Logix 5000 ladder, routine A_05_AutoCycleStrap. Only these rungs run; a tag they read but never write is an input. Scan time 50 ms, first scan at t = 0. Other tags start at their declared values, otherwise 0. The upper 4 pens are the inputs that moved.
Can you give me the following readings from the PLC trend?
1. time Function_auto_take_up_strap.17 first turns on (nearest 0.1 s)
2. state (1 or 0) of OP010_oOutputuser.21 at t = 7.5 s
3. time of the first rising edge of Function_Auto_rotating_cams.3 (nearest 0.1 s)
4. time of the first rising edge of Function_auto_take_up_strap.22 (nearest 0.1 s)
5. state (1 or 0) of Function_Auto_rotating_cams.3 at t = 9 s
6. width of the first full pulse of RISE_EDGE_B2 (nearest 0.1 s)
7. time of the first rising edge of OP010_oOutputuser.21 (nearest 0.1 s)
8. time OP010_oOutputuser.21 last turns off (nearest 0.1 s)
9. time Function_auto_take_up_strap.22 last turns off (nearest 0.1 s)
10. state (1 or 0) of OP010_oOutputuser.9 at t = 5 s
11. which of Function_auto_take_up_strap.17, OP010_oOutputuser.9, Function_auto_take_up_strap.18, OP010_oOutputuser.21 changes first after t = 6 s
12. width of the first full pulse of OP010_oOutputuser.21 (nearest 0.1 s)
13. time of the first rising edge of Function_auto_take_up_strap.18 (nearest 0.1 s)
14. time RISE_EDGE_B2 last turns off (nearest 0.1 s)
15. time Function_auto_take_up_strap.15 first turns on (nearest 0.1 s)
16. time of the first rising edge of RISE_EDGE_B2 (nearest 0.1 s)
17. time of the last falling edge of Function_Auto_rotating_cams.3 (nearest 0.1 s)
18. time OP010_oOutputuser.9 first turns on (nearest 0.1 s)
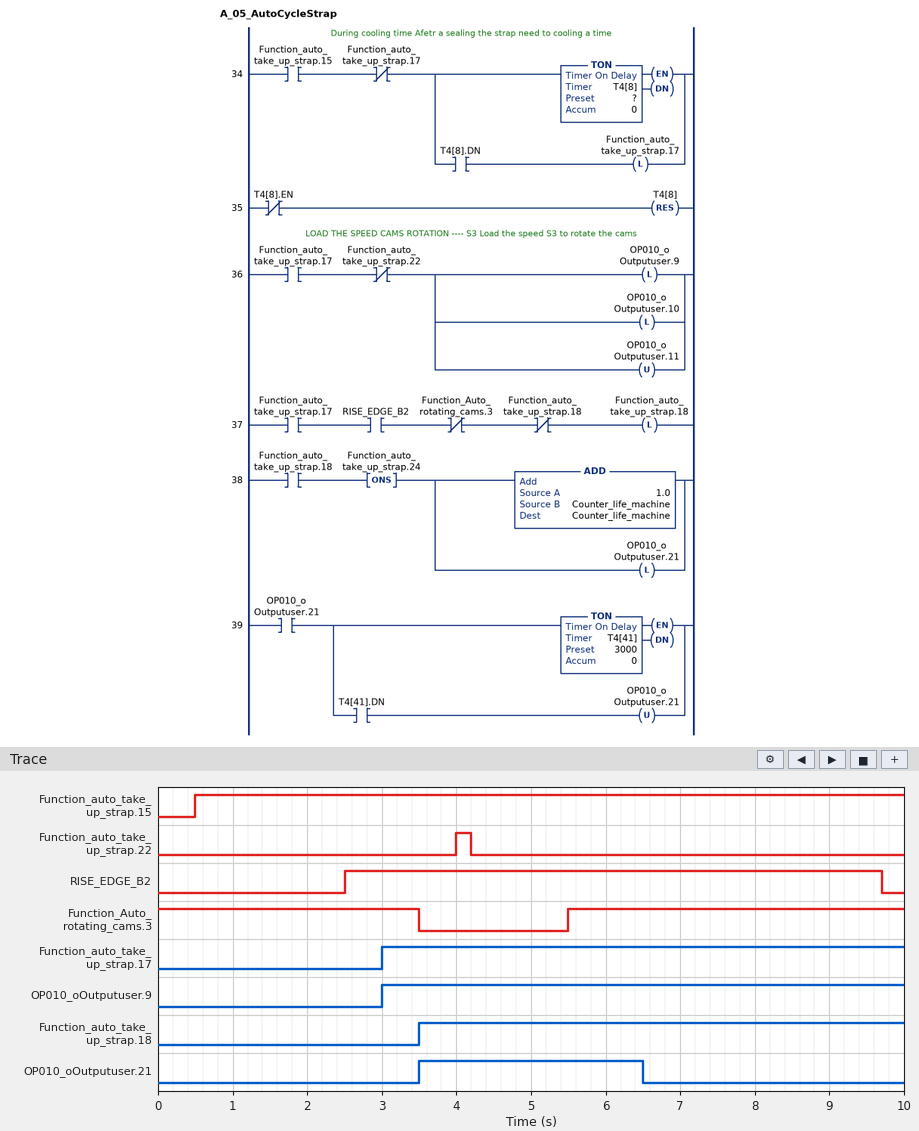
3.0 s
0
5.5 s
4.0 s
1
7.2 s
3.5 s
6.5 s
4.2 s
1
OP010_oOutputuser.21
3.0 s
3.5 s
9.7 s
0.5 s
2.5 s
3.5 s
3.0 s
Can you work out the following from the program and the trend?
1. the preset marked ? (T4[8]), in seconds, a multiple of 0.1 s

2.5 s
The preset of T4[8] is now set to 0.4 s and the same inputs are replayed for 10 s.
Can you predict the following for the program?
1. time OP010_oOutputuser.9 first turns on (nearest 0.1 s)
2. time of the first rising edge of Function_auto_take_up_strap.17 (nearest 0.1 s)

0.9 s
0.9 s
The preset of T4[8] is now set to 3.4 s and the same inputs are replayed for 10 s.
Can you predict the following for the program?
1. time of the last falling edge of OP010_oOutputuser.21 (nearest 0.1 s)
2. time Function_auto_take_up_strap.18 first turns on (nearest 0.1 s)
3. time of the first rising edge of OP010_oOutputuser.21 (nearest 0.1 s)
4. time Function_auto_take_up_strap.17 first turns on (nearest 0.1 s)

6.9 s
3.9 s
3.9 s
3.9 s
